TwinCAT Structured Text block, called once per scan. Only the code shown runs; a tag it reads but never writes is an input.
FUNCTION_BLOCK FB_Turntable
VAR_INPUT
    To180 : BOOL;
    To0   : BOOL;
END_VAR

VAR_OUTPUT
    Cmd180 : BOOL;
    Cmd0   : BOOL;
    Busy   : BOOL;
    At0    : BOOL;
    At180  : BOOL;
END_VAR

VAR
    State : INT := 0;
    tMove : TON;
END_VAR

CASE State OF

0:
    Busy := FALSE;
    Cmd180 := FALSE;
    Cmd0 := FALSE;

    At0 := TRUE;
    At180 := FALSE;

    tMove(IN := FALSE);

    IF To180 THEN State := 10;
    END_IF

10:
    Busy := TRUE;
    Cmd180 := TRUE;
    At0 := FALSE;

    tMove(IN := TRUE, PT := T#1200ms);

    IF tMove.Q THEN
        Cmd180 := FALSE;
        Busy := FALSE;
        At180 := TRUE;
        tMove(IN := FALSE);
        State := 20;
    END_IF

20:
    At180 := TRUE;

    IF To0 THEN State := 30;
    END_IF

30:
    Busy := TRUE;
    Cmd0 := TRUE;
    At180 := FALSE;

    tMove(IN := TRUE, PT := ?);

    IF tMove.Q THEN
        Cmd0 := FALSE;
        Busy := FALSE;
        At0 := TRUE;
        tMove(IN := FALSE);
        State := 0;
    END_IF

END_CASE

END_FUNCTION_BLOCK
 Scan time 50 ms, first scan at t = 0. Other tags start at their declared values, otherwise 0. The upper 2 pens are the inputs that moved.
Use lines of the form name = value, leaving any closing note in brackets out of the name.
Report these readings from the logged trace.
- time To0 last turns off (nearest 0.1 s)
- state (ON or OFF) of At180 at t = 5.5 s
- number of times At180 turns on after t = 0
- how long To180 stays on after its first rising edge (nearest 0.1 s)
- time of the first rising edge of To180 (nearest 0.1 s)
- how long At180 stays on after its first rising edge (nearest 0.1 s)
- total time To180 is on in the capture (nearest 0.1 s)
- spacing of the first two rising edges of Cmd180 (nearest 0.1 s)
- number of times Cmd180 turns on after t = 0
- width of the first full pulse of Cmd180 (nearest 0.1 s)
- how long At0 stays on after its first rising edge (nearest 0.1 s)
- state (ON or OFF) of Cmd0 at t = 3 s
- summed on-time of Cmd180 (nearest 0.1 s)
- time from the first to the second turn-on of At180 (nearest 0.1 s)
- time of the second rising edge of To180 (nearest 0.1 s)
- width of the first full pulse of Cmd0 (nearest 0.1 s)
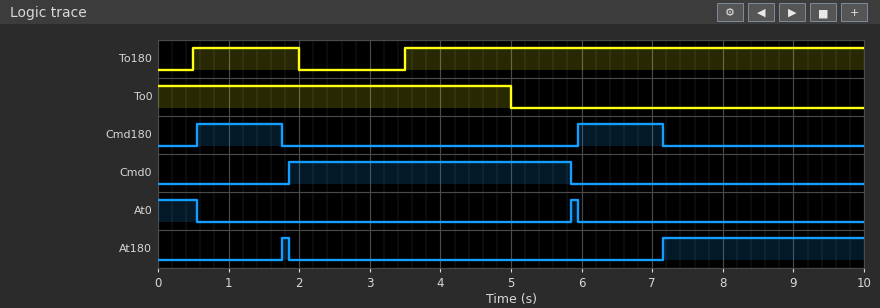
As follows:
time To0 last turns off = 5.0 s
state (ON or OFF) of At180 at t = 5.5 s = OFF
number of times At180 turns on after t = 0 = 2
how long To180 stays on after its first rising edge = 1.5 s
time of the first rising edge of To180 = 0.5 s
how long At180 stays on after its first rising edge = 0.1 s
total time To180 is on in the capture = 8.0 s
spacing of the first two rising edges of Cmd180 = 5.4 s
number of times Cmd180 turns on after t = 0 = 2
width of the first full pulse of Cmd180 = 1.2 s
how long At0 stays on after its first rising edge = 0.1 s
state (ON or OFF) of Cmd0 at t = 3 s = ON
summed on-time of Cmd180 = 2.4 s
time from the first to the second turn-on of At180 = 5.4 s
time of the second rising edge of To180 = 3.5 s
width of the first full pulse of Cmd0 = 4.0 s
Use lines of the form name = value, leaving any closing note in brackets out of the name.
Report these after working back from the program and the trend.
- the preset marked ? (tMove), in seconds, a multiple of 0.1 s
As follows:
the preset marked ? (tMove), in seconds, a multiple of 0.1 s = 4.0 s
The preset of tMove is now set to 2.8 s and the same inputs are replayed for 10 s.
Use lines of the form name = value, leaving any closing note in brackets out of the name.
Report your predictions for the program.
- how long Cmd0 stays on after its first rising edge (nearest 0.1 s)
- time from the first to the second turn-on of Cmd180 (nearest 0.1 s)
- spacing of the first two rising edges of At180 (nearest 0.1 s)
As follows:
how long Cmd0 stays on after its first rising edge = 2.8 s
time from the first to the second turn-on of Cmd180 = 4.2 s
spacing of the first two rising edges of At180 = 4.2 s
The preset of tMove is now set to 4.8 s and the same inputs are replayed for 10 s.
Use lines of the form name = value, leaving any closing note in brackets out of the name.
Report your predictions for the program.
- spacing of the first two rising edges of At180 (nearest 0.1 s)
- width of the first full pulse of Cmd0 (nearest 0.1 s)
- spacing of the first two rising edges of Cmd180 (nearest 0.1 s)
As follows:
spacing of the first two rising edges of At180 = 6.2 s
width of the first full pulse of Cmd0 = 4.8 s
spacing of the first two rising edges of Cmd180 = 6.2 s
